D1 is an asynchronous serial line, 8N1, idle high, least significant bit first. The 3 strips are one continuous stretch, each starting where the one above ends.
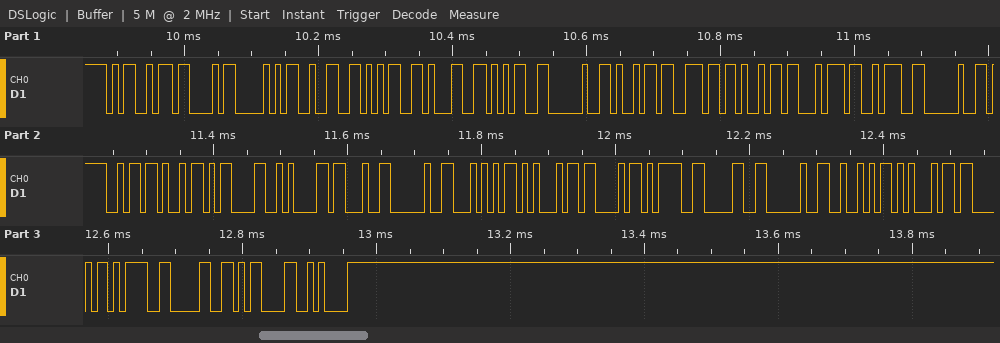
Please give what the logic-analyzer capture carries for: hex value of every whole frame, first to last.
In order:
4D 43 50 32 35 31 35 20 69 6E 69 74 3A 20 4F 4B 0D 0A 23 20 54 45 43 3D 30 20 52 45 43 3D 30 0D 0A
